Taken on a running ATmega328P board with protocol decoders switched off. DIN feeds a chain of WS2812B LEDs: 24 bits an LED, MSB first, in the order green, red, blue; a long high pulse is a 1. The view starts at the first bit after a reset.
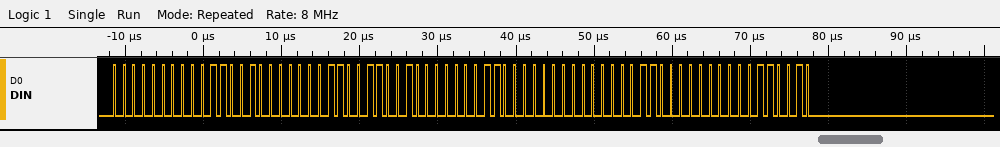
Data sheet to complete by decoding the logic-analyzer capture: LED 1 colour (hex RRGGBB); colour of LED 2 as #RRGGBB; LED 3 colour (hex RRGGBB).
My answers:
#320003
#033200
#000332
